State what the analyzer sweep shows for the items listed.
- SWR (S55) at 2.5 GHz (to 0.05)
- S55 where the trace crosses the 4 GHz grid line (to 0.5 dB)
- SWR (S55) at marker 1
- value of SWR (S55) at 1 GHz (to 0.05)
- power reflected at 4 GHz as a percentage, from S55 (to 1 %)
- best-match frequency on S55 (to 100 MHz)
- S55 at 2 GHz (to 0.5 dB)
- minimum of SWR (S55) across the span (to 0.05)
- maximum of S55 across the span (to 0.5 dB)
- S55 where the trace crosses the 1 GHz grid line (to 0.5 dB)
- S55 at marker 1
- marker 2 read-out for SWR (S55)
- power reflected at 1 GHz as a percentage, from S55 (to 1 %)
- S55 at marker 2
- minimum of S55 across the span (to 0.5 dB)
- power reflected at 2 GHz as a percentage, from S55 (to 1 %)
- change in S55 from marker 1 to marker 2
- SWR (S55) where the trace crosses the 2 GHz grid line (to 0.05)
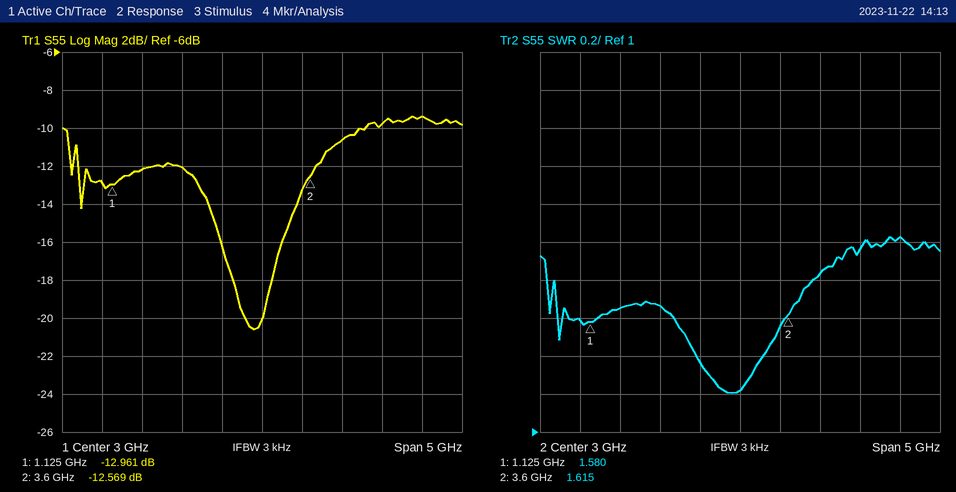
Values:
1.35
-10.5 dB
1.580
1.60
9 %
2.9 GHz
-12.0 dB
1.20
-9.5 dB
-13.0 dB
-12.961 dB
1.615
5 %
-12.569 dB
-20.5 dB
6 %
0.392 dB
1.65
